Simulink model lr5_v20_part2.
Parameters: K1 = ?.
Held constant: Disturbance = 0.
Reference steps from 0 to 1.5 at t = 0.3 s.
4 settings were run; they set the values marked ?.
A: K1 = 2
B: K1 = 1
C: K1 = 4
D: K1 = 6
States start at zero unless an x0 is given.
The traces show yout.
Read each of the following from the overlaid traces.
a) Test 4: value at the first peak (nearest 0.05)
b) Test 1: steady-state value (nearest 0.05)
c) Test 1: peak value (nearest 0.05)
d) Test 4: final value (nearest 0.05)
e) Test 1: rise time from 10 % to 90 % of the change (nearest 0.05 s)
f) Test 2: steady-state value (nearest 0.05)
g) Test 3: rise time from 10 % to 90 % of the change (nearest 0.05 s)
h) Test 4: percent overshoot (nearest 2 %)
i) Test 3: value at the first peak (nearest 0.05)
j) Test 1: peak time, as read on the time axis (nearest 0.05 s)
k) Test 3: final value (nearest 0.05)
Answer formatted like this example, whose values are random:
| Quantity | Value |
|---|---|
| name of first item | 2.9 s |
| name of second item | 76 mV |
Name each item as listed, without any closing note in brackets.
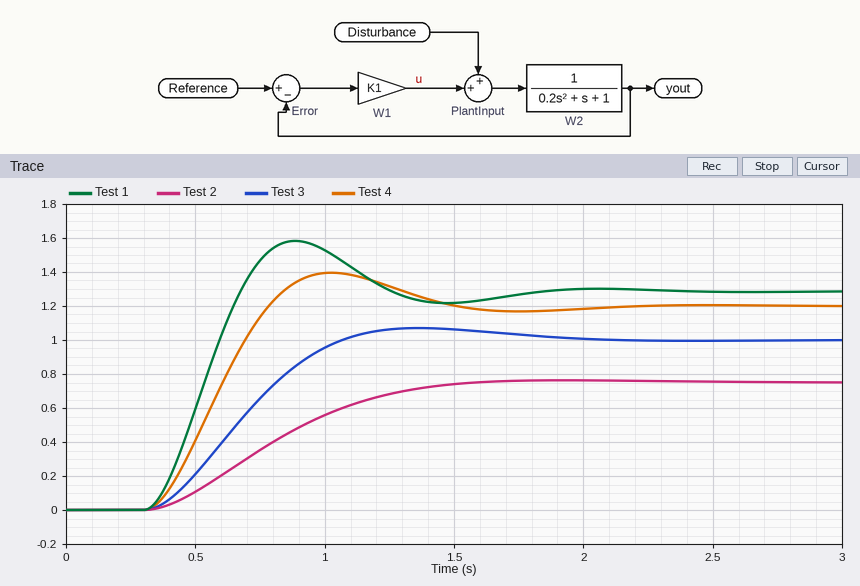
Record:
| Quantity | Value |
|---|---|
| Test 4: value at the first peak | 1.40 |
| Test 1: steady-state value | 1.30 |
| Test 1: peak value | 1.60 |
| Test 4: final value | 1.20 |
| Test 1: rise time from 10 % to 90 % of the change | 0.25 s |
| Test 2: steady-state value | 0.75 |
| Test 3: rise time from 10 % to 90 % of the change | 0.50 s |
| Test 4: percent overshoot | 16 % |
| Test 3: value at the first peak | 1.05 |
| Test 1: peak time, as read on the time axis | 0.90 s |
| Test 3: final value | 1.00 |
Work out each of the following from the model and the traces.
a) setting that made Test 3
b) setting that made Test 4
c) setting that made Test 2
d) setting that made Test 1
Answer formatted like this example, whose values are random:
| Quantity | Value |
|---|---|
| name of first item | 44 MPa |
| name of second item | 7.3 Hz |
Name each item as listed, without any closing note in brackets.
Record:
| Quantity | Value |
|---|---|
| setting that made Test 3 | A |
| setting that made Test 4 | C |
| setting that made Test 2 | B |
| setting that made Test 1 | D |
